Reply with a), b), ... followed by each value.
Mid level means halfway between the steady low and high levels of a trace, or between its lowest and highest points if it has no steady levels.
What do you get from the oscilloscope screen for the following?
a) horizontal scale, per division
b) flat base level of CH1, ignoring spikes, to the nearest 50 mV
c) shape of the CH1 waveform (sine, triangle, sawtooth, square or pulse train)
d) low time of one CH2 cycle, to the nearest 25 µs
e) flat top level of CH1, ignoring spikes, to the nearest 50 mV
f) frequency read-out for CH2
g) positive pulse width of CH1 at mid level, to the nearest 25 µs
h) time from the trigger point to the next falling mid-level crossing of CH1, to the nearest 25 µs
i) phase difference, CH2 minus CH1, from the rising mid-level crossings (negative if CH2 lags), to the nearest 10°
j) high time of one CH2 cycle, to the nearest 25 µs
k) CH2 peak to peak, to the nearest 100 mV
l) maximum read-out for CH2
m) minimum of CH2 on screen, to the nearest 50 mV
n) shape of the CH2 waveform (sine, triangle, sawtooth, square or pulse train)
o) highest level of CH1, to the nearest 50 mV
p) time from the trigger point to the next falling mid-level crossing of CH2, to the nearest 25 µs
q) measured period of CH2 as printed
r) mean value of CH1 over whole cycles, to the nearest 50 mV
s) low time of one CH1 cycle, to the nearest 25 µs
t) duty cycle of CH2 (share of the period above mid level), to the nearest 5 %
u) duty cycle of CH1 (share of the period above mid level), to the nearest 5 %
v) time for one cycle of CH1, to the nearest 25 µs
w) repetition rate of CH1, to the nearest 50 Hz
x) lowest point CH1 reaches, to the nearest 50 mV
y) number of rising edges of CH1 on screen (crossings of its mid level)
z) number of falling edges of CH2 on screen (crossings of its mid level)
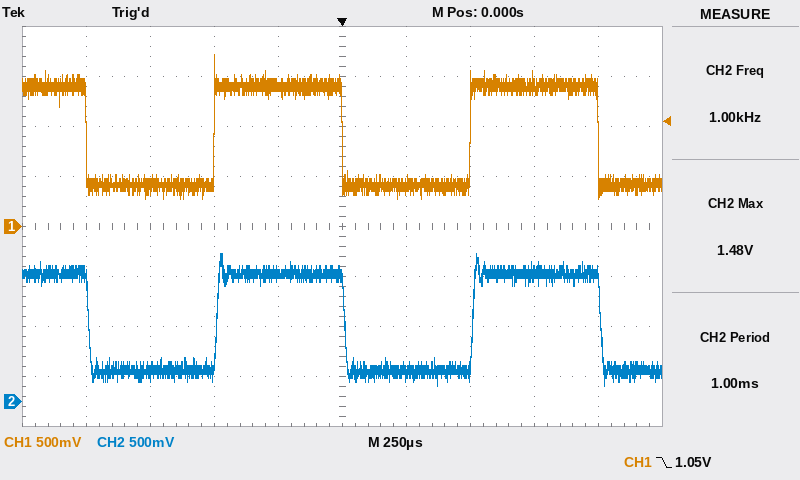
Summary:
a) 250 µs
b) 400 mV
c) square
d) 500 µs
e) 1.40 V
f) 1.00 kHz
g) 500 µs
h) 1.000 ms
i) 0°
j) 500 µs
k) 1.30 V
l) 1.48 V
m) 150 mV
n) square
o) 1.70 V
p) 1.000 ms
q) 1.00 ms
r) 900 mV
s) 500 µs
t) 50 %
u) 50 %
v) 1.000 ms
w) 1.00 kHz
x) 300 mV
y) 2
z) 3
